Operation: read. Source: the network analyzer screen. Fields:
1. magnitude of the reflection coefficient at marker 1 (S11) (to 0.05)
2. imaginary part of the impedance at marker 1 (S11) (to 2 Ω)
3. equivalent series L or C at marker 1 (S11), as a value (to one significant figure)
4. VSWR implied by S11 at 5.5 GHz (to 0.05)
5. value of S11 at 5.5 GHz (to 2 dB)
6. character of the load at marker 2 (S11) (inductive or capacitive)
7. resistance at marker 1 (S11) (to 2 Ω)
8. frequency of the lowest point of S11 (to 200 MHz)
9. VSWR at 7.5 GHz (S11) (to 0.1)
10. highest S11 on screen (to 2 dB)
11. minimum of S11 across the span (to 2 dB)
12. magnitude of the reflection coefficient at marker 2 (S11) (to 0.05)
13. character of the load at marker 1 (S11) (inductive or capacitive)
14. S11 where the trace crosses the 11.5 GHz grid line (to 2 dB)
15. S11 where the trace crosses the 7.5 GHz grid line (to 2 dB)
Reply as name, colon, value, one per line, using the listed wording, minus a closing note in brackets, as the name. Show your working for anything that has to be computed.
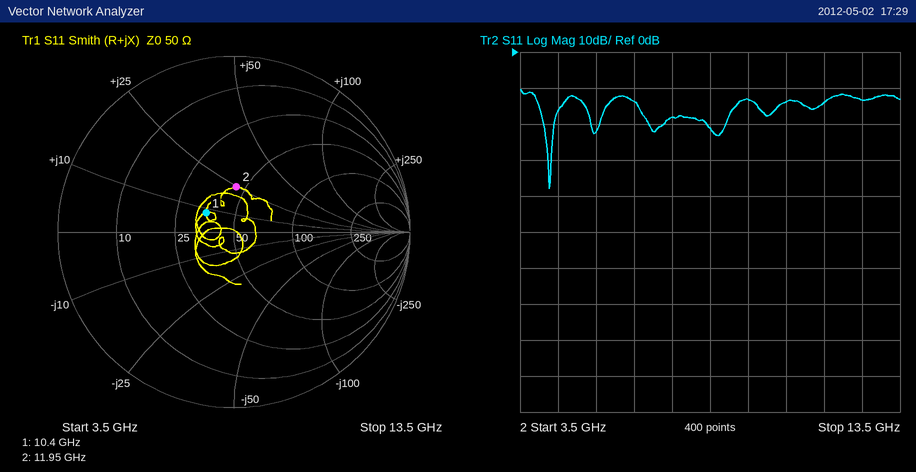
magnitude of the reflection coefficient at marker 1 (S11): 0.20
imaginary part of the impedance at marker 1 (S11): +8 Ω
equivalent series L or C at marker 1 (S11), as a value: L = 8 Ω/(2π × 10.4 GHz) ≈ 122 pH, so 100 pH to one significant figure
VSWR implied by S11 at 5.5 GHz: |Γ| = 10^(-22/20) = 0.0794; VSWR = (1 + 0.0794)/(1 − 0.0794) ≈ 1.17, so 1.15 to the nearest 0.05
value of S11 at 5.5 GHz: -22 dB
character of the load at marker 2 (S11): inductive
resistance at marker 1 (S11): 36 Ω
frequency of the lowest point of S11: 4.2 GHz
VSWR at 7.5 GHz (S11): |Γ| = 10^(-18/20) = 0.1259; VSWR = (1 + 0.1259)/(1 − 0.1259) ≈ 1.3
highest S11 on screen: -10 dB
minimum of S11 across the span: -38 dB
magnitude of the reflection coefficient at marker 2 (S11): 0.25
character of the load at marker 1 (S11): inductive
S11 where the trace crosses the 11.5 GHz grid line: -14 dB
S11 where the trace crosses the 7.5 GHz grid line: -18 dB
